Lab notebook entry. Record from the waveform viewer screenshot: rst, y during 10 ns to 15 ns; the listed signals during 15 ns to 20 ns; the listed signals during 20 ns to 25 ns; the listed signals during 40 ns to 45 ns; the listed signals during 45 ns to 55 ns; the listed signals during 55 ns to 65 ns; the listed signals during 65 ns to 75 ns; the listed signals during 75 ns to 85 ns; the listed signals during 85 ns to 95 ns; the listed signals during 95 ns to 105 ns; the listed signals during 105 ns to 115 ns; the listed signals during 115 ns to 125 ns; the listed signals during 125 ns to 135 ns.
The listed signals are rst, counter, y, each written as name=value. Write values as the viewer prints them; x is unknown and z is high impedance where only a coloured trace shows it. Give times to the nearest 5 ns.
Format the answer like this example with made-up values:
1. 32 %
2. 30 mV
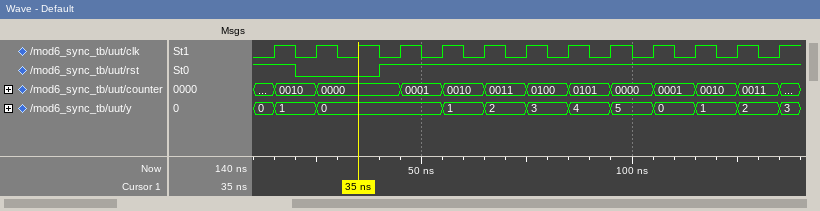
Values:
1. rst=1, y=0
2. rst=1, counter=0010, y=1
3. rst=0, counter=0010, y=1
4. rst=1, counter=0000, y=0
5. rst=1, counter=0001, y=0
6. rst=1, counter=0010, y=1
7. rst=1, counter=0011, y=2
8. rst=1, counter=0100, y=3
9. rst=1, counter=0101, y=4
10. rst=1, counter=0000, y=5
11. rst=1, counter=0001, y=0
12. rst=1, counter=0010, y=1
13. rst=1, counter=0011, y=2
